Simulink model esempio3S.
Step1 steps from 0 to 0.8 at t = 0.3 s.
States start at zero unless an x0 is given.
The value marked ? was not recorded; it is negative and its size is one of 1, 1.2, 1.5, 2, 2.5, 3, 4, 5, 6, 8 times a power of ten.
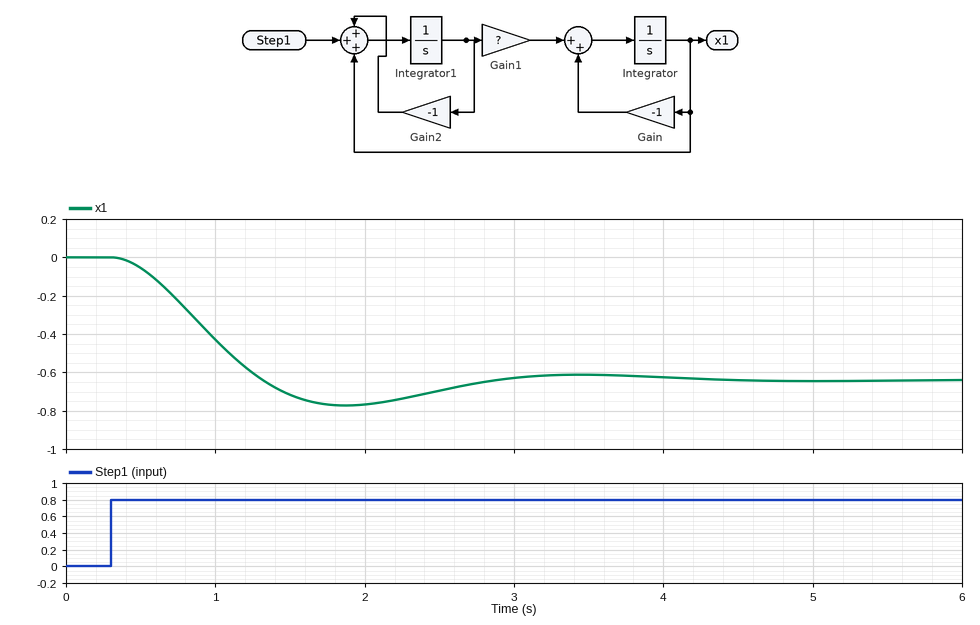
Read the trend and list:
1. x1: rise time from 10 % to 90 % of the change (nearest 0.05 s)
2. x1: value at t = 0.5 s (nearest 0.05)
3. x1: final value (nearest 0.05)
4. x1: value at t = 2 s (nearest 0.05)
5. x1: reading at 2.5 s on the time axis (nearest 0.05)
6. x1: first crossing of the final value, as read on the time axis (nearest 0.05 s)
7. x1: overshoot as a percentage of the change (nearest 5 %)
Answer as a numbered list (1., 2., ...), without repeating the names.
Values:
1. 0.70 s
2. -0.05
3. -0.65
4. -0.75
5. -0.70
6. 1.30 s
7. 20 %
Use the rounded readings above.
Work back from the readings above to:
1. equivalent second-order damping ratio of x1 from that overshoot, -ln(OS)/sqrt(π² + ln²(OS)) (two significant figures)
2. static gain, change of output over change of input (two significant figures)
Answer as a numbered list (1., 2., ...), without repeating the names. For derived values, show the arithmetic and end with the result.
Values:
1. ln(0.2) = -1.609; 1.609 / sqrt(9.870 + 2.590) = 0.46
2. (-0.65 - 0) / (0.8 - 0) = -0.81
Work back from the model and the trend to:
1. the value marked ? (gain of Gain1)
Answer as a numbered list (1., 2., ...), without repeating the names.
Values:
1. -4
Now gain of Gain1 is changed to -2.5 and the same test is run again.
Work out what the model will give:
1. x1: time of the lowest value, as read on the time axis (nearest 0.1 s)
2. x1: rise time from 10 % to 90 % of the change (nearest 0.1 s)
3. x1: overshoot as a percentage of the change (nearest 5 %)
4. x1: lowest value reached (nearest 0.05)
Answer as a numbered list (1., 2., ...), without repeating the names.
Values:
1. 2.3 s
2. 0.9 s
3. 15 %
4. -0.65
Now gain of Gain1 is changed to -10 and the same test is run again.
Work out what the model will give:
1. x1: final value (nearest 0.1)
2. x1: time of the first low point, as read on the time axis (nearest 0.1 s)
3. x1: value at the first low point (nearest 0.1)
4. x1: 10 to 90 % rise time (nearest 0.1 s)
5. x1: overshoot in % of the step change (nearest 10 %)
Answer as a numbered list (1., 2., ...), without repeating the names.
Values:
1. -0.7
2. 1.3 s
3. -1.0
4. 0.4 s
5. 40 %
